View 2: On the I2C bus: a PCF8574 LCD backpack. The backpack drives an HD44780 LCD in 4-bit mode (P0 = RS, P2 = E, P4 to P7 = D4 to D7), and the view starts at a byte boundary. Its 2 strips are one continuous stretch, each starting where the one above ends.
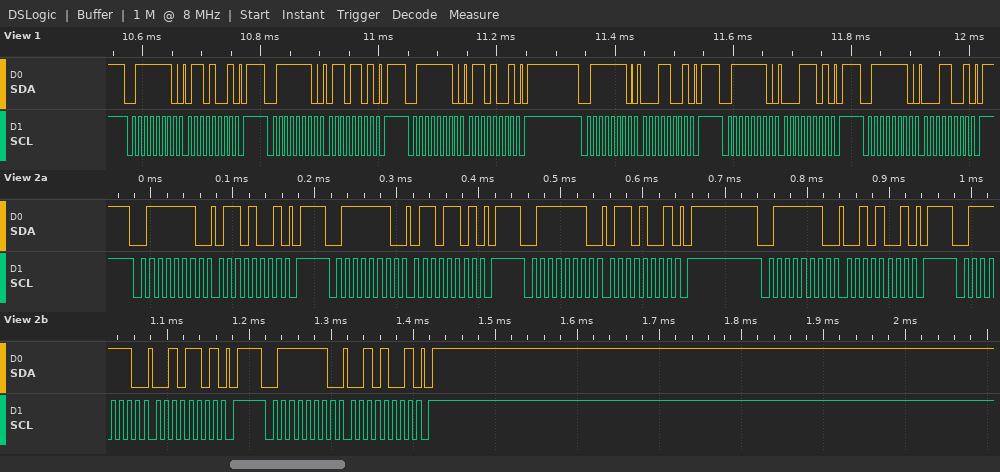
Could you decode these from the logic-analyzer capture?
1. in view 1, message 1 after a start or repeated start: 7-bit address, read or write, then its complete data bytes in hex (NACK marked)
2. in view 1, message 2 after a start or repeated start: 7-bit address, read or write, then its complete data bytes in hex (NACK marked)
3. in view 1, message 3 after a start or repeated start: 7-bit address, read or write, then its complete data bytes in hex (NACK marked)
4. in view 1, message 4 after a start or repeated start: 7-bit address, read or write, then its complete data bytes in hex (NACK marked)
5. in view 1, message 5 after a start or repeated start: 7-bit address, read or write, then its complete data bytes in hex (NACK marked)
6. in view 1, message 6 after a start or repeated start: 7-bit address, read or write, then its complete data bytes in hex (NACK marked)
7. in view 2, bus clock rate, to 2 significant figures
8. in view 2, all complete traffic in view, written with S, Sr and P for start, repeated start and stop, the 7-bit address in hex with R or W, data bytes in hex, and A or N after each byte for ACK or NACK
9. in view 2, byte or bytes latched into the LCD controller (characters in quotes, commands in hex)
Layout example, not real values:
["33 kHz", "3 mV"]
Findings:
["0x3F write: 69", "0x3F write: 6D", "0x3F write: 69", "0x3F write: 19", "0x3F write: 1D", "0x3F write: 19", "100 kHz", "S 3FW A 69 A P S 3FW A 6D A P S 3FW A 69 A P S 3FW A 29 A P S 3FW A 2D A P S 3FW A 29 A P", "'b'"]
